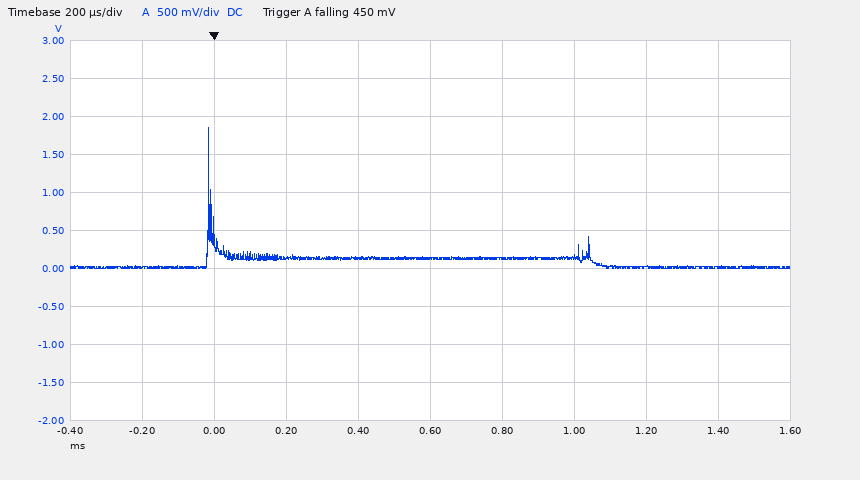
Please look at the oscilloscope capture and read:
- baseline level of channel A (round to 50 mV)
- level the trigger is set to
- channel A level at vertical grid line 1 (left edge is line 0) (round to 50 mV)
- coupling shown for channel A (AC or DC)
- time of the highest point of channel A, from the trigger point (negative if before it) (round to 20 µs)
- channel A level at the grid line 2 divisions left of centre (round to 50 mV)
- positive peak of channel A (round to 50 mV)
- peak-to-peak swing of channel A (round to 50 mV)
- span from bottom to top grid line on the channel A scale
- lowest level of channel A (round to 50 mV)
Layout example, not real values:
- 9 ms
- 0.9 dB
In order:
- 150 mV
- 450 mV
- 0 mV
- DC
- -20 µs
- 150 mV
- 1.85 V
- 1.85 V
- 5 V
- 0 mV
